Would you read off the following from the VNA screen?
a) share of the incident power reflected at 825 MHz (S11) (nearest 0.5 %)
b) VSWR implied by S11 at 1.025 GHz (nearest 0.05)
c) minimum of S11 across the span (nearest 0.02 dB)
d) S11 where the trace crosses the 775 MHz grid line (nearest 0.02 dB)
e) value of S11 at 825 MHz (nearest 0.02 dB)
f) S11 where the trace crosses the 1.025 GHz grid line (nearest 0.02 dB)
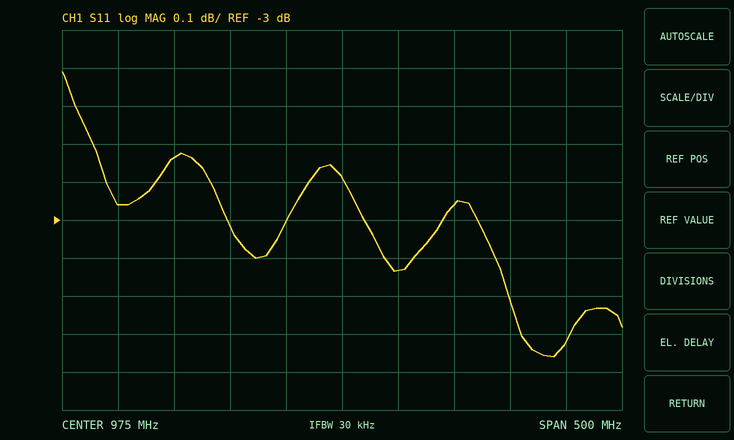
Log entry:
52.0 %
5.60
-3.36 dB
-2.96 dB
-2.84 dB
-3.14 dB
